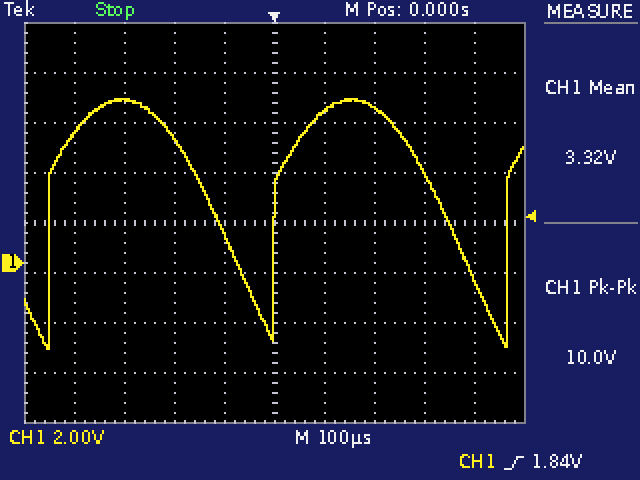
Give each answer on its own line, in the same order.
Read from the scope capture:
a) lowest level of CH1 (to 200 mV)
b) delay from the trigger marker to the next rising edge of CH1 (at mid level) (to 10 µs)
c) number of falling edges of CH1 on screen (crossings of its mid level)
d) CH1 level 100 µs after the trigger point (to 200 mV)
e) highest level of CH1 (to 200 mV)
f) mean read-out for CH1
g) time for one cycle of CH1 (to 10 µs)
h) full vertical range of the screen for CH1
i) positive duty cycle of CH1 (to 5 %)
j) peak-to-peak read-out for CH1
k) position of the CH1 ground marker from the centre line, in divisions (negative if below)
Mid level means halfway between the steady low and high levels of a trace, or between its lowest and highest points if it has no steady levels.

-3.4 V
470 µs
2
6.0 V
6.6 V
3.32 V
460 µs
16 V
75 %
10.0 V
-0.8 div
